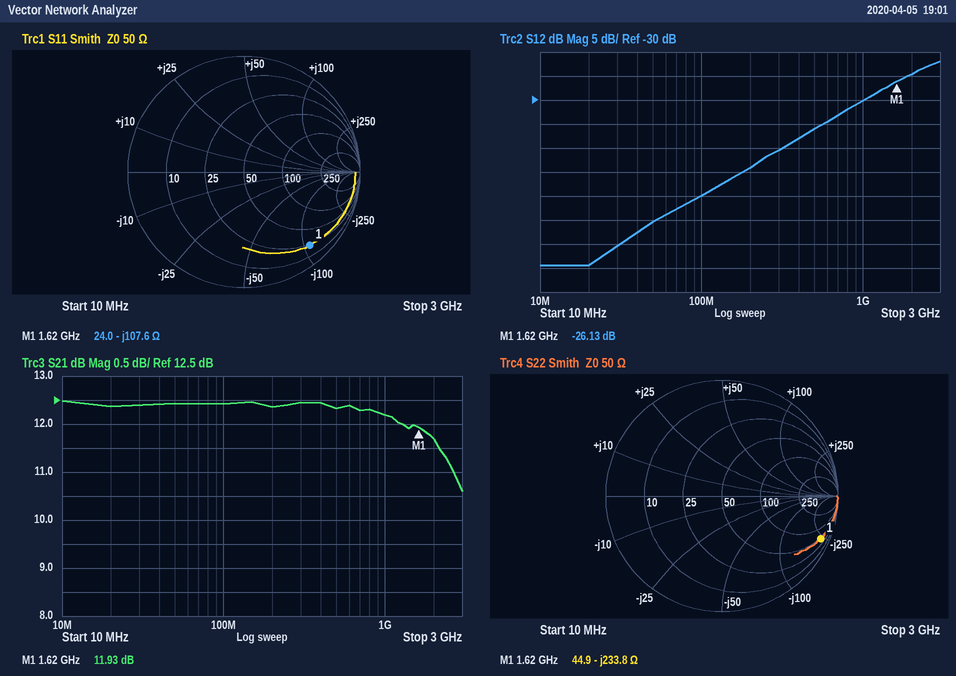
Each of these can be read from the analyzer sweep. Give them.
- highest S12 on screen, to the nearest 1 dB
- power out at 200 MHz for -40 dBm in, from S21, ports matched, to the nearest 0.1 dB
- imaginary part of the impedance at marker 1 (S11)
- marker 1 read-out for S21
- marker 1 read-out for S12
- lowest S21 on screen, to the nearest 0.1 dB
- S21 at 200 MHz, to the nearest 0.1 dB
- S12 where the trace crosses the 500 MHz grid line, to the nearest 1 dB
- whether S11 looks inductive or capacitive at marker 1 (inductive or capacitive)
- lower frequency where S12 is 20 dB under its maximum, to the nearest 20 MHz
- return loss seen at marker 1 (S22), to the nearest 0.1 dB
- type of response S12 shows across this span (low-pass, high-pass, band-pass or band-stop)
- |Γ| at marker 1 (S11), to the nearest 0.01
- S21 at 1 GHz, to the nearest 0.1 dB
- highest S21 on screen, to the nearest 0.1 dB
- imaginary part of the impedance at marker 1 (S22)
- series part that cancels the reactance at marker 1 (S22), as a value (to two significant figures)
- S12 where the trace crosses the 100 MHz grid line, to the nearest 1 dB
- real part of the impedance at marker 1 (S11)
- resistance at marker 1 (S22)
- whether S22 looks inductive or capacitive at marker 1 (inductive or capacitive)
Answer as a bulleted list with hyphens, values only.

- -22 dB
- -27.6 dBm
- -107.6 Ω
- 11.93 dB
- -26.13 dB
- 10.6 dB
- 12.4 dB
- -36 dB
- capacitive
- 240 MHz
- 0.7 dB
- high-pass
- 0.85
- 12.2 dB
- 12.5 dB
- -233.8 Ω
- 23 nH
- -50 dB
- 24.0 Ω
- 44.9 Ω
- capacitive
